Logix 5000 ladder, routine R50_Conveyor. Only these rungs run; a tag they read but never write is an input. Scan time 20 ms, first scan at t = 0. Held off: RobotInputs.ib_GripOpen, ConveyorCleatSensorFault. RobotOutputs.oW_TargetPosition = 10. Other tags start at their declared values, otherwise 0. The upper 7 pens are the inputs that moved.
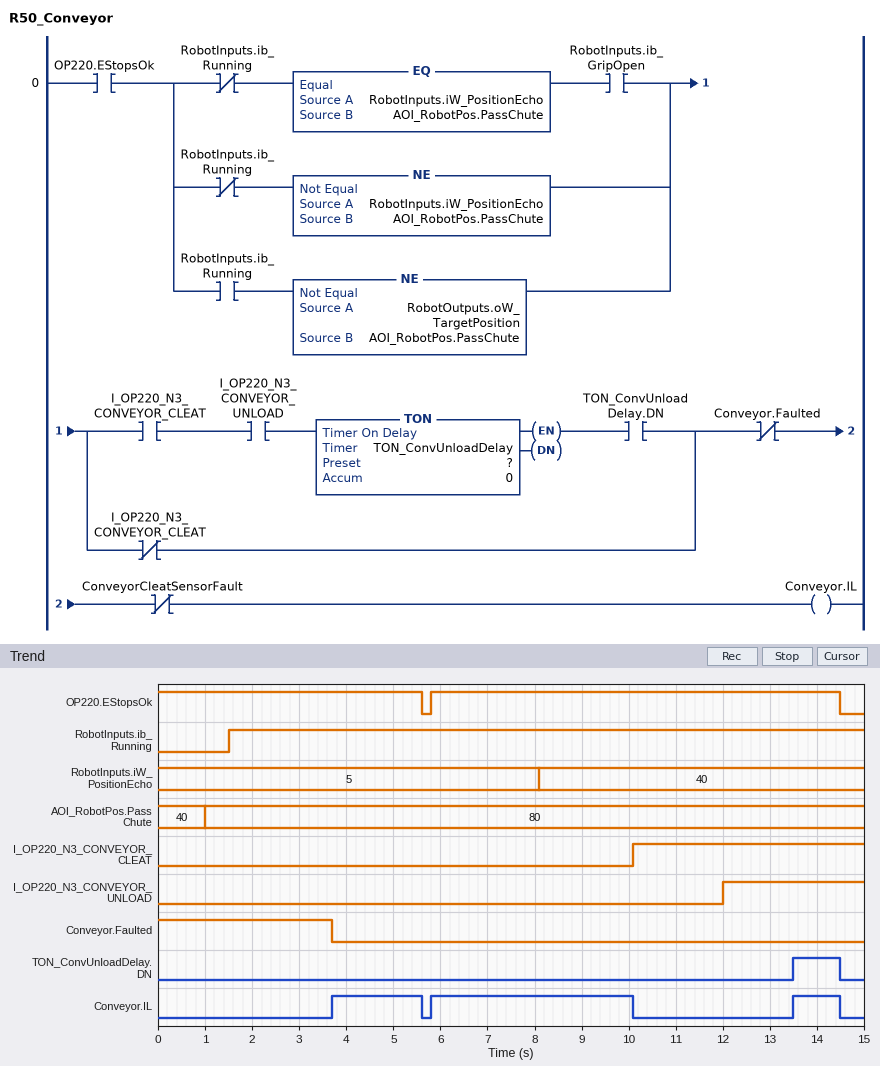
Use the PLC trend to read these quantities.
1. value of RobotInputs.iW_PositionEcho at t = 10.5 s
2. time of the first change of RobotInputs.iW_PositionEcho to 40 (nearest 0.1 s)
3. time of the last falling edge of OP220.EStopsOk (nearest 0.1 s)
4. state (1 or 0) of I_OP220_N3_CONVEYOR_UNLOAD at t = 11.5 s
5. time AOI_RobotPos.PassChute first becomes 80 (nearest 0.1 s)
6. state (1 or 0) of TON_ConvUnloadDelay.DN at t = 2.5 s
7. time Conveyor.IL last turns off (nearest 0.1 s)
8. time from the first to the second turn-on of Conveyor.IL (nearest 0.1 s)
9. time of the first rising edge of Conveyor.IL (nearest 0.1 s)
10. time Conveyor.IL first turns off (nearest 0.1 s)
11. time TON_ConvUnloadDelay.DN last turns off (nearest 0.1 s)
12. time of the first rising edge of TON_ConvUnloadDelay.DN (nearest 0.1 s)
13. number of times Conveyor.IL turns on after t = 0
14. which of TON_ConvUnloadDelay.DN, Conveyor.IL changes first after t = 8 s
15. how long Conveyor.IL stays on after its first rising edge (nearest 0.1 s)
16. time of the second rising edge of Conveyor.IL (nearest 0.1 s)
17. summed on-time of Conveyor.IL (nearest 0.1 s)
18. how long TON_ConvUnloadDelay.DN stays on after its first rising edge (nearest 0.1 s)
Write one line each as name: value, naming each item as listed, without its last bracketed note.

value of RobotInputs.iW_PositionEcho at t = 10.5 s: 40
time of the first change of RobotInputs.iW_PositionEcho to 40: 8.1 s
time of the last falling edge of OP220.EStopsOk: 14.5 s
state (1 or 0) of I_OP220_N3_CONVEYOR_UNLOAD at t = 11.5 s: 0
time AOI_RobotPos.PassChute first becomes 80: 1.0 s
state (1 or 0) of TON_ConvUnloadDelay.DN at t = 2.5 s: 0
time Conveyor.IL last turns off: 14.5 s
time from the first to the second turn-on of Conveyor.IL: 2.1 s
time of the first rising edge of Conveyor.IL: 3.7 s
time Conveyor.IL first turns off: 5.6 s
time TON_ConvUnloadDelay.DN last turns off: 14.5 s
time of the first rising edge of TON_ConvUnloadDelay.DN: 13.5 s
number of times Conveyor.IL turns on after t = 0: 3
which of TON_ConvUnloadDelay.DN, Conveyor.IL changes first after t = 8 s: Conveyor.IL
how long Conveyor.IL stays on after its first rising edge: 1.9 s
time of the second rising edge of Conveyor.IL: 5.8 s
summed on-time of Conveyor.IL: 7.2 s
how long TON_ConvUnloadDelay.DN stays on after its first rising edge: 1.0 s
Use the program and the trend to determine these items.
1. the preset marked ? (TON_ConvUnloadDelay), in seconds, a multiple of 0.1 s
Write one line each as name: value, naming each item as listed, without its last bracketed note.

the preset marked ? (TON_ConvUnloadDelay), in seconds, a multiple of 0.1 s: 1.5 s
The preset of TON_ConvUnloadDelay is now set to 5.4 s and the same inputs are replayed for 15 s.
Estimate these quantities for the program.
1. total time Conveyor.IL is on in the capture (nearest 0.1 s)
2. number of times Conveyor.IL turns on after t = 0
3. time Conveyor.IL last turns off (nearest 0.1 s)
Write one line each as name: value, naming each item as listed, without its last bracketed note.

total time Conveyor.IL is on in the capture: 6.2 s
number of times Conveyor.IL turns on after t = 0: 2
time Conveyor.IL last turns off: 10.1 s
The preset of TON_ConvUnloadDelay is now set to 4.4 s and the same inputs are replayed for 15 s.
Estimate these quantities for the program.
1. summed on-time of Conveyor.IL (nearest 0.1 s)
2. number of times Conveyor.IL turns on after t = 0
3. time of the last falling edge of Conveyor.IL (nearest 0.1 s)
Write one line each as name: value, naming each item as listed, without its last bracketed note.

summed on-time of Conveyor.IL: 6.2 s
number of times Conveyor.IL turns on after t = 0: 2
time of the last falling edge of Conveyor.IL: 10.1 s
